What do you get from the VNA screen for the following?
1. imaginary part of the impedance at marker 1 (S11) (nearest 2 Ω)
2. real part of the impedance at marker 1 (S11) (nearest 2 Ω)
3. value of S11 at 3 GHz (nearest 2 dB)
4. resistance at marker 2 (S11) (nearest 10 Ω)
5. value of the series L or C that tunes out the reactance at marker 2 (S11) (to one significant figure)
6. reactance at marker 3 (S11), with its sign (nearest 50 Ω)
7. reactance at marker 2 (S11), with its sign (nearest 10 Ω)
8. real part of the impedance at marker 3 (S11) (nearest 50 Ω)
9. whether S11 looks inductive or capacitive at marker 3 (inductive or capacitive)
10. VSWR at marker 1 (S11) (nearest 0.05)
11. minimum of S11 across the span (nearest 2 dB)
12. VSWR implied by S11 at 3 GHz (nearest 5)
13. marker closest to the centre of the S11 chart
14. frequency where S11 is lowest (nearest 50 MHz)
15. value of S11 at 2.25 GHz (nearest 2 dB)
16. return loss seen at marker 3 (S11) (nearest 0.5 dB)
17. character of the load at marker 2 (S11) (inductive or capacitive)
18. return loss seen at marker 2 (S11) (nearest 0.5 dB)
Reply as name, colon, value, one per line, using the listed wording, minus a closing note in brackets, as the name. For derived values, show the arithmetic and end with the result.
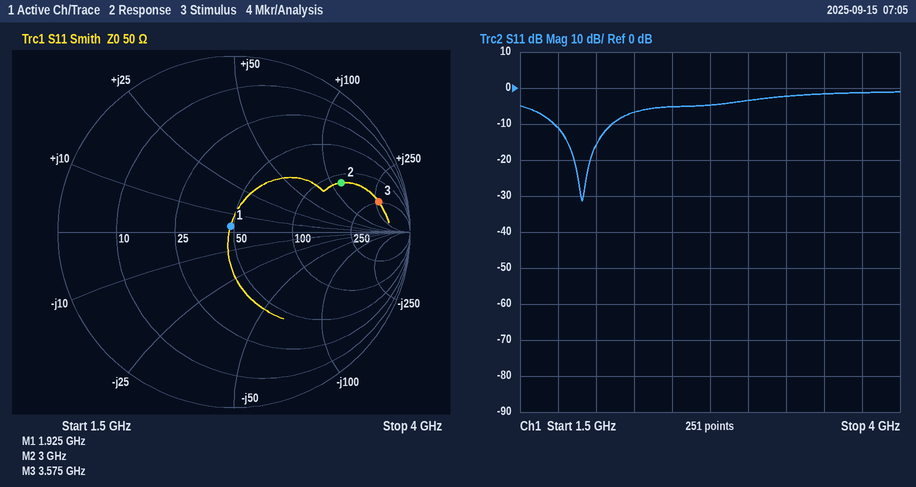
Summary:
imaginary part of the impedance at marker 1 (S11): +4 Ω
real part of the impedance at marker 1 (S11): 48 Ω
value of S11 at 3 GHz: -4 dB
resistance at marker 2 (S11): 120 Ω
value of the series L or C that tunes out the reactance at marker 2 (S11): C = 1/(2π × 3 GHz × 120 Ω) ≈ 442 fF, so 400 fF to one significant figure
reactance at marker 3 (S11), with its sign: +300 Ω
reactance at marker 2 (S11), with its sign: +120 Ω
real part of the impedance at marker 3 (S11): 250 Ω
whether S11 looks inductive or capacitive at marker 3: inductive
VSWR at marker 1 (S11): 1.10
minimum of S11 across the span: -32 dB
VSWR implied by S11 at 3 GHz: |Γ| = 10^(-4/20) = 0.6310; VSWR = (1 + 0.6310)/(1 − 0.6310) ≈ 4.42, so 5 to the nearest 5
marker closest to the centre of the S11 chart: marker 1
frequency where S11 is lowest: 1.90 GHz
value of S11 at 2.25 GHz: -6 dB
return loss seen at marker 3 (S11): 1.5 dB
character of the load at marker 2 (S11): inductive
return loss seen at marker 2 (S11): 3.5 dB
